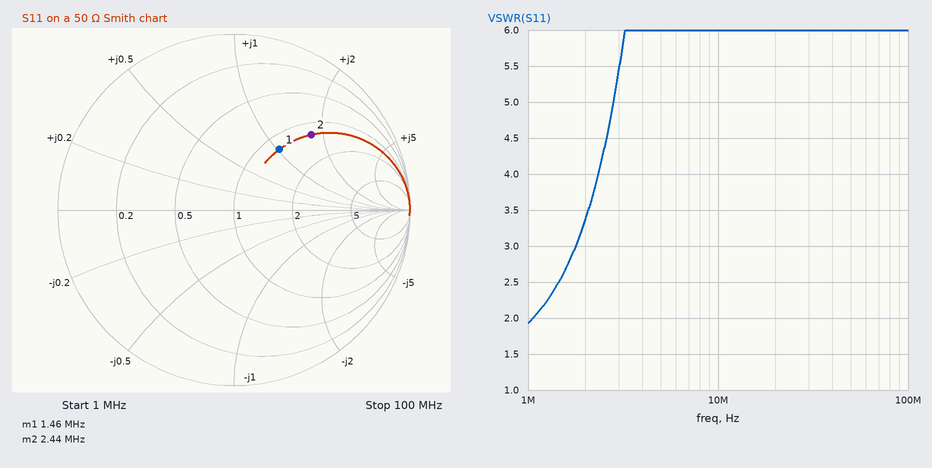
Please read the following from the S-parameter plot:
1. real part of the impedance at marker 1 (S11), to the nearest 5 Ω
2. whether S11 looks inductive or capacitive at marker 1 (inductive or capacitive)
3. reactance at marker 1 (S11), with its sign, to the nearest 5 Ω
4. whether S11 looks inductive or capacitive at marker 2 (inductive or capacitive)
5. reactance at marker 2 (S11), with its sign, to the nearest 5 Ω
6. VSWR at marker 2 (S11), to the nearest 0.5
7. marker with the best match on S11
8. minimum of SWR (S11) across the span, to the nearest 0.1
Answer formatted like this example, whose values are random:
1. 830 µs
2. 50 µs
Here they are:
1. 60 Ω
2. inductive
3. +50 Ω
4. inductive
5. +85 Ω
6. 4.0
7. marker 1
8. 1.9
